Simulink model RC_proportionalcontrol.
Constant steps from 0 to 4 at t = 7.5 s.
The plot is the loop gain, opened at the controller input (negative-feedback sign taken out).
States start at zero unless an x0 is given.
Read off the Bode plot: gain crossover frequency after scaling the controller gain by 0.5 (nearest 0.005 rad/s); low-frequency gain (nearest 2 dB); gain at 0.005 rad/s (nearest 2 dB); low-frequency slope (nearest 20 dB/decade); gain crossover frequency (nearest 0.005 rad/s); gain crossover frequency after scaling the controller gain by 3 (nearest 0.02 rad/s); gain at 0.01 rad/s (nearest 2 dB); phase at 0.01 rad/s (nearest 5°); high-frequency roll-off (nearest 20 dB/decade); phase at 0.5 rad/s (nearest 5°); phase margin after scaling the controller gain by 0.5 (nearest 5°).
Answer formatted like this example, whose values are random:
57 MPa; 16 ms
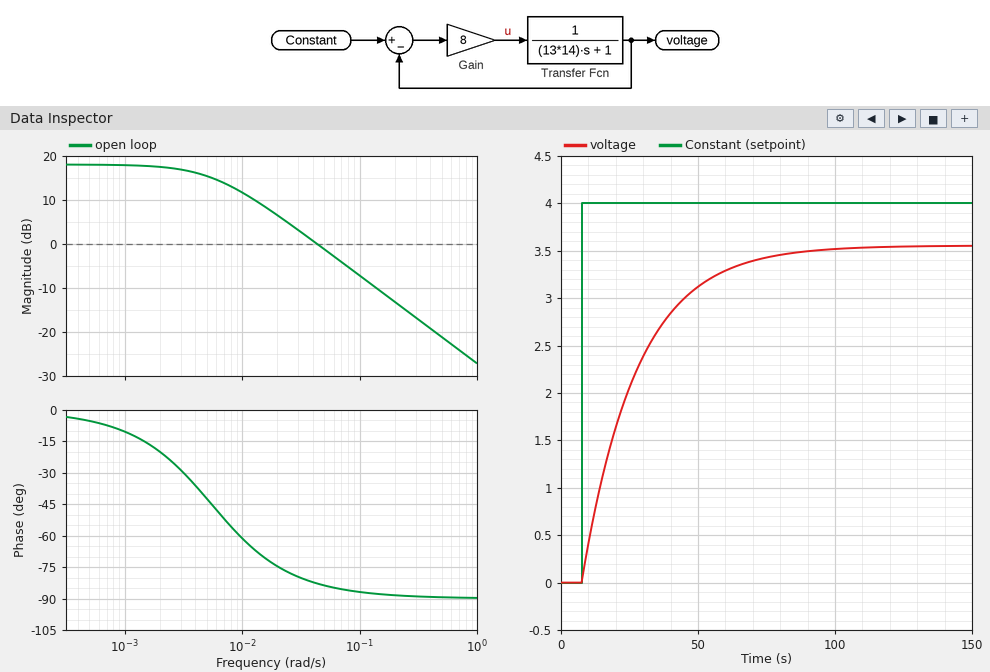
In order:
0.020 rad/s; 18 dB; 16 dB; 0 dB/decade; 0.045 rad/s; 0.14 rad/s; 12 dB; -60°; -20 dB/decade; -90°; 105°
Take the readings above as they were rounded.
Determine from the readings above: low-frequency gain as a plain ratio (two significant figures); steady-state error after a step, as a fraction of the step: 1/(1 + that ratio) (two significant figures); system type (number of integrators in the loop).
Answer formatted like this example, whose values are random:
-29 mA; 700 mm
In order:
7.9; 0.11; 0
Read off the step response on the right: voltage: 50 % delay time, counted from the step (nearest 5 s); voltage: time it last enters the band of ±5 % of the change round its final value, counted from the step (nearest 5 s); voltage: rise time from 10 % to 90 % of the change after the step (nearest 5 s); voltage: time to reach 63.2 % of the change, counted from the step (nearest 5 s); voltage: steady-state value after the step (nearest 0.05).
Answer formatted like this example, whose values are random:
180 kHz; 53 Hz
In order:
15 s; 60 s; 45 s; 20 s; 3.55
